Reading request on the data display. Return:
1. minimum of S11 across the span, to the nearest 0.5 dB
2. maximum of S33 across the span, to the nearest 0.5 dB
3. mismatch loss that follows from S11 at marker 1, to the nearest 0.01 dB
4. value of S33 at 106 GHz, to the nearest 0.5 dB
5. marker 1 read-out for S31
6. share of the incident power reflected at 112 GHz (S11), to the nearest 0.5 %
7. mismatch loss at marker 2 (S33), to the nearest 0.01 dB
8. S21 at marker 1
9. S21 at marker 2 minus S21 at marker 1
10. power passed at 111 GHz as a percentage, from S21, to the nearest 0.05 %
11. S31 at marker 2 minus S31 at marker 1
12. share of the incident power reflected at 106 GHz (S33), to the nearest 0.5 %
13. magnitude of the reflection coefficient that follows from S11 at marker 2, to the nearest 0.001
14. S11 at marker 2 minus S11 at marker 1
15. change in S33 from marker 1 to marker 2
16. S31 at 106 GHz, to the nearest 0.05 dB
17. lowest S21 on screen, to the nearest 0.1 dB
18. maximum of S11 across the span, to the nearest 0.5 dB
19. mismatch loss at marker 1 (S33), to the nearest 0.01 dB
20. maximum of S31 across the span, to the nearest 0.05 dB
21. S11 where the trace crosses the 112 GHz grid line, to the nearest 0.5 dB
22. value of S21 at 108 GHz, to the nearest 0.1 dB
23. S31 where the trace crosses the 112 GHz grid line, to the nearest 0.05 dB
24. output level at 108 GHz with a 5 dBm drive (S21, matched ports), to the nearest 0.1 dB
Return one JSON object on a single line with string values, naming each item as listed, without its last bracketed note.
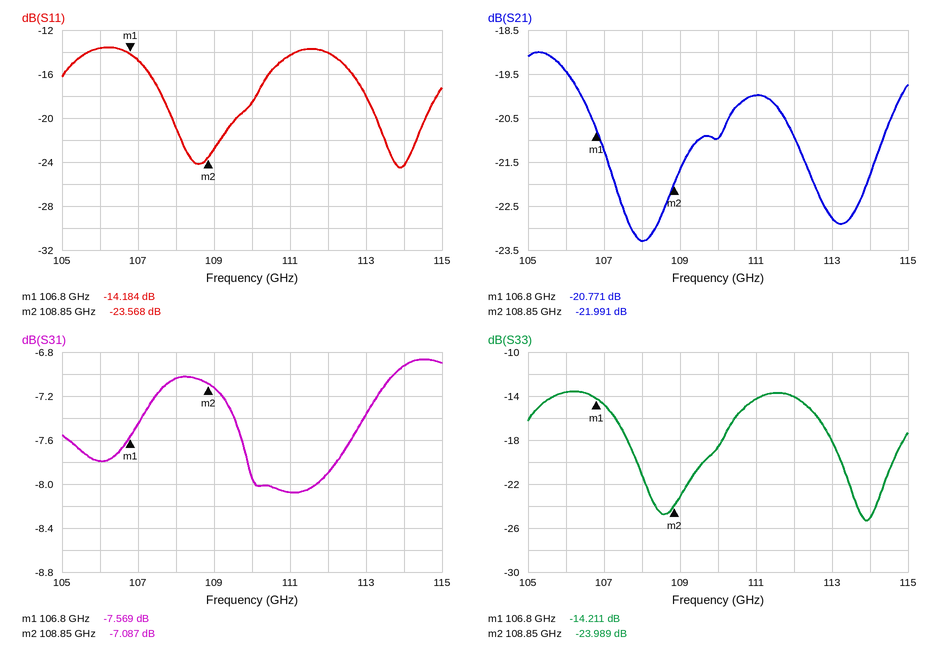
{"minimum of S11 across the span, to the nearest 0.5 dB": "-24.5 dB", "maximum of S33 across the span, to the nearest 0.5 dB": "-13.5 dB", "mismatch loss that follows from S11 at marker 1, to the nearest 0.01 dB": "0.17 dB", "value of S33 at 106 GHz, to the nearest 0.5 dB": "-13.5 dB", "marker 1 read-out for S31": "-7.569 dB", "share of the incident power reflected at 112 GHz (S11), to the nearest 0.5 %": "4.0 %", "mismatch loss at marker 2 (S33), to the nearest 0.01 dB": "0.02 dB", "S21 at marker 1": "-20.771 dB", "S21 at marker 2 minus S21 at marker 1": "-1.220 dB", "power passed at 111 GHz as a percentage, from S21, to the nearest 0.05 %": "1.00 %", "S31 at marker 2 minus S31 at marker 1": "0.482 dB", "share of the incident power reflected at 106 GHz (S33), to the nearest 0.5 %": "4.5 %", "magnitude of the reflection coefficient that follows from S11 at marker 2, to the nearest 0.001": "0.066", "S11 at marker 2 minus S11 at marker 1": "-9.384 dB", "change in S33 from marker 1 to marker 2": "-9.778 dB", "S31 at 106 GHz, to the nearest 0.05 dB": "-7.80 dB", "lowest S21 on screen, to the nearest 0.1 dB": "-23.3 dB", "maximum of S11 across the span, to the nearest 0.5 dB": "-13.5 dB", "mismatch loss at marker 1 (S33), to the nearest 0.01 dB": "0.17 dB", "maximum of S31 across the span, to the nearest 0.05 dB": "-6.85 dB", "S11 where the trace crosses the 112 GHz grid line, to the nearest 0.5 dB": "-14.0 dB", "value of S21 at 108 GHz, to the nearest 0.1 dB": "-23.3 dB", "S31 where the trace crosses the 112 GHz grid line, to the nearest 0.05 dB": "-7.90 dB", "output level at 108 GHz with a 5 dBm drive (S21, matched ports), to the nearest 0.1 dB": "-18.3 dBm"}
